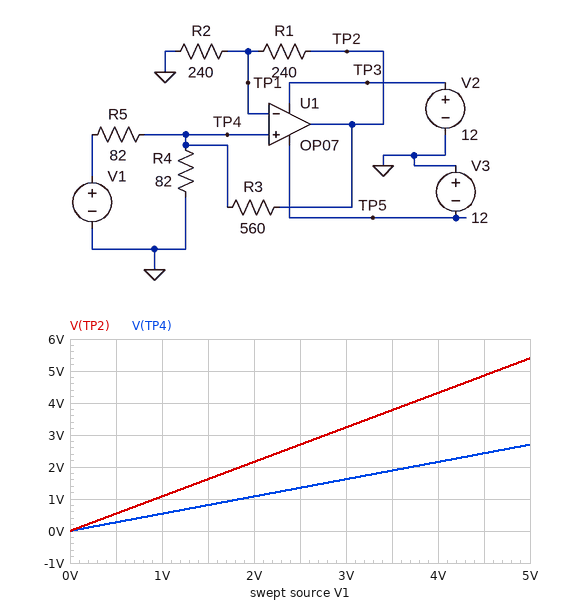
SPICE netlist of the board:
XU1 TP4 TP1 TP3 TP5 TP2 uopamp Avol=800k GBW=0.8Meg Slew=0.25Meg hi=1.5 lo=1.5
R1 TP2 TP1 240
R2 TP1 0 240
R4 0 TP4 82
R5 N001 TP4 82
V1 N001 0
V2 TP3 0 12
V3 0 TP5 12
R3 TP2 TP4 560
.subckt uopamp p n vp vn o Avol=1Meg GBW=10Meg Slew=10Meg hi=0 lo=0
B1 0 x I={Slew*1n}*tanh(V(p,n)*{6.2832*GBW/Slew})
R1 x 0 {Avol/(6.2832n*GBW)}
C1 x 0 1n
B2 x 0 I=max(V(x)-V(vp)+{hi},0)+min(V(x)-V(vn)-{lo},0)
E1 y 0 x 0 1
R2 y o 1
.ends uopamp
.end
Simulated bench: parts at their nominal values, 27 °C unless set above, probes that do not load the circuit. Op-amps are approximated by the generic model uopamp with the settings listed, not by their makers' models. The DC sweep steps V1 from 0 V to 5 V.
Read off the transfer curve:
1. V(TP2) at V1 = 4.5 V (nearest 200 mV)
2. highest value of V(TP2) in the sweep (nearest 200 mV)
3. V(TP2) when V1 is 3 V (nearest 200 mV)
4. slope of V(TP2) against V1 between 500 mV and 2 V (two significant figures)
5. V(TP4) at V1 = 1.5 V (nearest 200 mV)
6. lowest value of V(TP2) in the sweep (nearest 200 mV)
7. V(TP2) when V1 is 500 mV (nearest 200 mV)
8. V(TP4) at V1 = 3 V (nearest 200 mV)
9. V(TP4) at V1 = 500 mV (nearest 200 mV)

4.8 V
5.4 V
3.2 V
1.1 V/V
800 mV
0 V
600 mV
1.6 V
200 mV
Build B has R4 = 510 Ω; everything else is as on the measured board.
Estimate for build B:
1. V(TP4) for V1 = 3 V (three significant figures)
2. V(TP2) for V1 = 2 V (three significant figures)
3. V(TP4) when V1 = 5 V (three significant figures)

2.96 V
3.94 V
4.93 V
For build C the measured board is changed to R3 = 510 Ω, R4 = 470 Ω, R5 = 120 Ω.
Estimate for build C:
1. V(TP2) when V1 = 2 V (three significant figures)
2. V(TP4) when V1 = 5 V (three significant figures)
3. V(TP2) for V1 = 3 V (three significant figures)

3.92 V
4.90 V
5.88 V
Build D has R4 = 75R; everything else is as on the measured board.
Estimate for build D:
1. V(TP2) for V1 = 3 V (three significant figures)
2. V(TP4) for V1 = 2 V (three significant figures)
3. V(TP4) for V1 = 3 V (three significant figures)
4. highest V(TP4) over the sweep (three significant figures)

3.08 V
1.03 V
1.54 V
2.57 V
